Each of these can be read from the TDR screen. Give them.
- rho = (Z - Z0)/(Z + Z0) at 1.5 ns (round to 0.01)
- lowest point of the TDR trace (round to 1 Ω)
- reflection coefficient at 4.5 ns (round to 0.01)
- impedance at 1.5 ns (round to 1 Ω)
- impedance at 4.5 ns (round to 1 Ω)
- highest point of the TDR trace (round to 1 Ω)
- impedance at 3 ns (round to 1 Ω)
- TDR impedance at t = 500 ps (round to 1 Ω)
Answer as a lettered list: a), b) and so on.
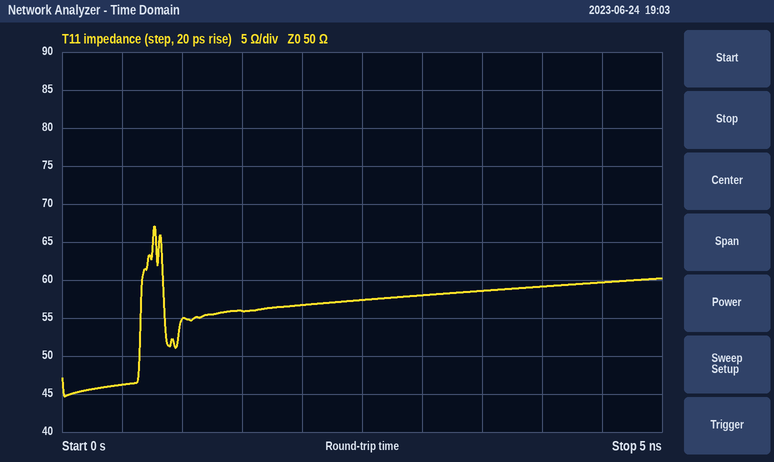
a) +0.06
b) 45 Ω
c) +0.09
d) 56 Ω
e) 60 Ω
f) 67 Ω
g) 58 Ω
h) 46 Ω
